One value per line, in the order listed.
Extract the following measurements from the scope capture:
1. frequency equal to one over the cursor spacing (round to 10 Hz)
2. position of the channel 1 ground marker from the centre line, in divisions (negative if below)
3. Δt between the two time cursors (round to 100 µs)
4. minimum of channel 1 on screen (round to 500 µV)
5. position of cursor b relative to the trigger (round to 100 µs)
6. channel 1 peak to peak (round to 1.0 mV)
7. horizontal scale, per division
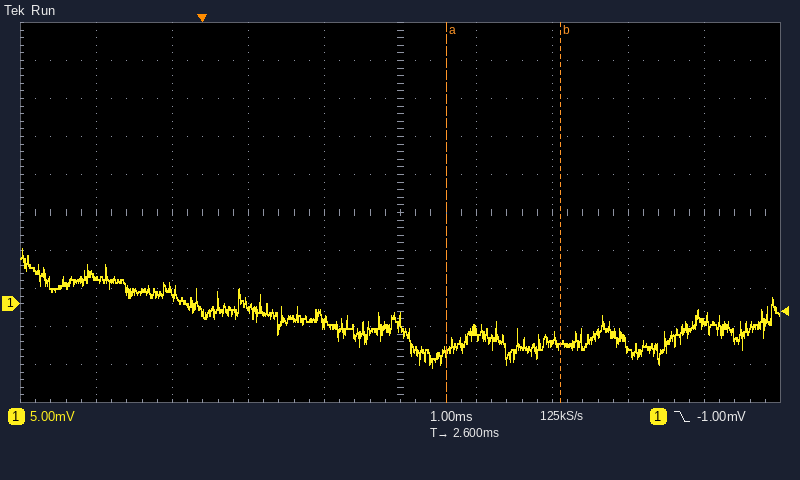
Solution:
670 Hz
-2.4 div
1.5 ms
-8.5 mV
+4.7 ms
16.0 mV
1 ms
